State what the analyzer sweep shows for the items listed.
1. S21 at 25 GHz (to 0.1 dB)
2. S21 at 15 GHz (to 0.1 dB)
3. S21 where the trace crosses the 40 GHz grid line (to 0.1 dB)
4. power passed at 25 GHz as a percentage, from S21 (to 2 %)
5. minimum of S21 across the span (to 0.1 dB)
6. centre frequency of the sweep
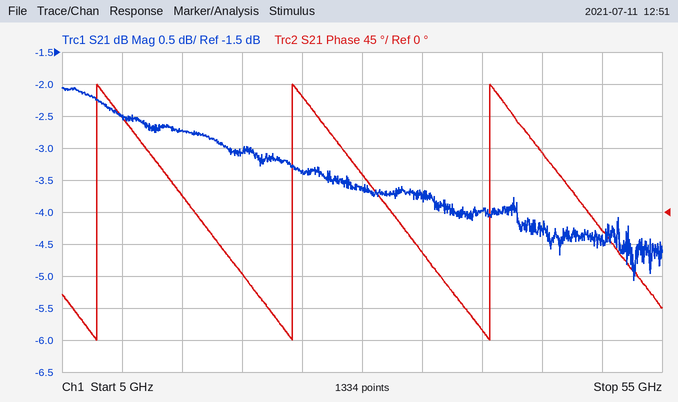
-3.4 dB
-2.7 dB
-4.0 dB
46 %
-5.1 dB
30 GHz
